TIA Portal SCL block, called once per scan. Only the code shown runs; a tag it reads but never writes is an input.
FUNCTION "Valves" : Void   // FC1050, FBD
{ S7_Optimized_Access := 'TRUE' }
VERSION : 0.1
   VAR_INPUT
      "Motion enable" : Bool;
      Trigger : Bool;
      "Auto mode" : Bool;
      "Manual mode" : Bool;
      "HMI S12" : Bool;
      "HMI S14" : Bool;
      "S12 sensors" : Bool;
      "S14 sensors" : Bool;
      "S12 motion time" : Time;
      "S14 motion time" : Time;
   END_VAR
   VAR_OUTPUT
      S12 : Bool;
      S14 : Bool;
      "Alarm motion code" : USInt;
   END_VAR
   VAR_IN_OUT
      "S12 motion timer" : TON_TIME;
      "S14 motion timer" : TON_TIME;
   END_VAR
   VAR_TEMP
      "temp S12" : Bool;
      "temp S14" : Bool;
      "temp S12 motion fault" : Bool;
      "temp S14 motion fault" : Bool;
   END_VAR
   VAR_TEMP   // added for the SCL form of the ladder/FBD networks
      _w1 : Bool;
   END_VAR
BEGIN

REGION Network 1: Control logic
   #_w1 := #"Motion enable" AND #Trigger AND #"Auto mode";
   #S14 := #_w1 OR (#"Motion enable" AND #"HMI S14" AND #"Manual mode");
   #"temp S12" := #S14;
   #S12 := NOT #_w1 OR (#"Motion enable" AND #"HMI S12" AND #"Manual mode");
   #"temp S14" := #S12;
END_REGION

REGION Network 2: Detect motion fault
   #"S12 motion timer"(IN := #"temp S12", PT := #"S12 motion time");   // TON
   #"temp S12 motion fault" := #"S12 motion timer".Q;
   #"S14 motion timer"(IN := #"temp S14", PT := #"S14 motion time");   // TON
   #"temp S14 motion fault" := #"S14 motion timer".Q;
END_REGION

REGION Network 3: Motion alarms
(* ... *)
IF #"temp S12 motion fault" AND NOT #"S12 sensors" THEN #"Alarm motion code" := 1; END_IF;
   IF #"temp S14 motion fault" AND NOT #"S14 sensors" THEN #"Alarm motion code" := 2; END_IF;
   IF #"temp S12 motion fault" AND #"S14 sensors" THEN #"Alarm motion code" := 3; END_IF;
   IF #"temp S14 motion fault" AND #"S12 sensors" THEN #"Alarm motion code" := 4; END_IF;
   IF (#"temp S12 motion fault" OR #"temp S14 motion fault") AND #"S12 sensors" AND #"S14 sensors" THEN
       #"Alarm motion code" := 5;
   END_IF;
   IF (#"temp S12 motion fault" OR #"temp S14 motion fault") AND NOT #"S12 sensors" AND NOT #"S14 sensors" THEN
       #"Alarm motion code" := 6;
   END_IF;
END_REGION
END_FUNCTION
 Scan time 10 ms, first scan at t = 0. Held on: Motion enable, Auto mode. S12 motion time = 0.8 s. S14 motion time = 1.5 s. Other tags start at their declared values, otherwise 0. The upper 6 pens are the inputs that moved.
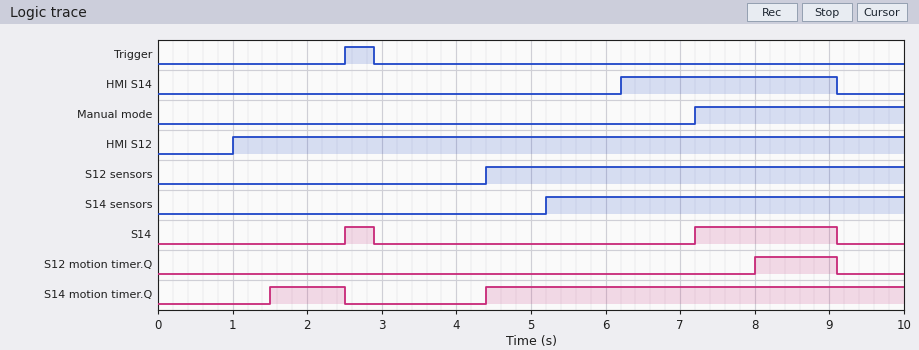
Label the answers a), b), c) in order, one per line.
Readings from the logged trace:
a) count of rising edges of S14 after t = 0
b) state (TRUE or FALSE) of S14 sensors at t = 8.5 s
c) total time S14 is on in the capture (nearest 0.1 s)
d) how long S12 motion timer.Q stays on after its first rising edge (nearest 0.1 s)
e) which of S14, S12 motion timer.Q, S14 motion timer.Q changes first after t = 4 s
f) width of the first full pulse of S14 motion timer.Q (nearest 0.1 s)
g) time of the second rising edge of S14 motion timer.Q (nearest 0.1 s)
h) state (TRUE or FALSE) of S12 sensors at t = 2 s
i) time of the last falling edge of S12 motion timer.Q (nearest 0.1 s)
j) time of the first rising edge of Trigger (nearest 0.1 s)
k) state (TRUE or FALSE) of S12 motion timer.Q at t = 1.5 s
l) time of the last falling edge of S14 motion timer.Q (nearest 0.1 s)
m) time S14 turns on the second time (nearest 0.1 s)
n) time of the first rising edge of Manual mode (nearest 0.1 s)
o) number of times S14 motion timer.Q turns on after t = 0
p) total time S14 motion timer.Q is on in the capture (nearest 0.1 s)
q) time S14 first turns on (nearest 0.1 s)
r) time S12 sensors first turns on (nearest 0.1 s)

a) 2
b) TRUE
c) 2.3 s
d) 1.1 s
e) S14 motion timer.Q
f) 1.0 s
g) 4.4 s
h) FALSE
i) 9.1 s
j) 2.5 s
k) FALSE
l) 2.5 s
m) 7.2 s
n) 7.2 s
o) 2
p) 6.6 s
q) 2.5 s
r) 4.4 s
